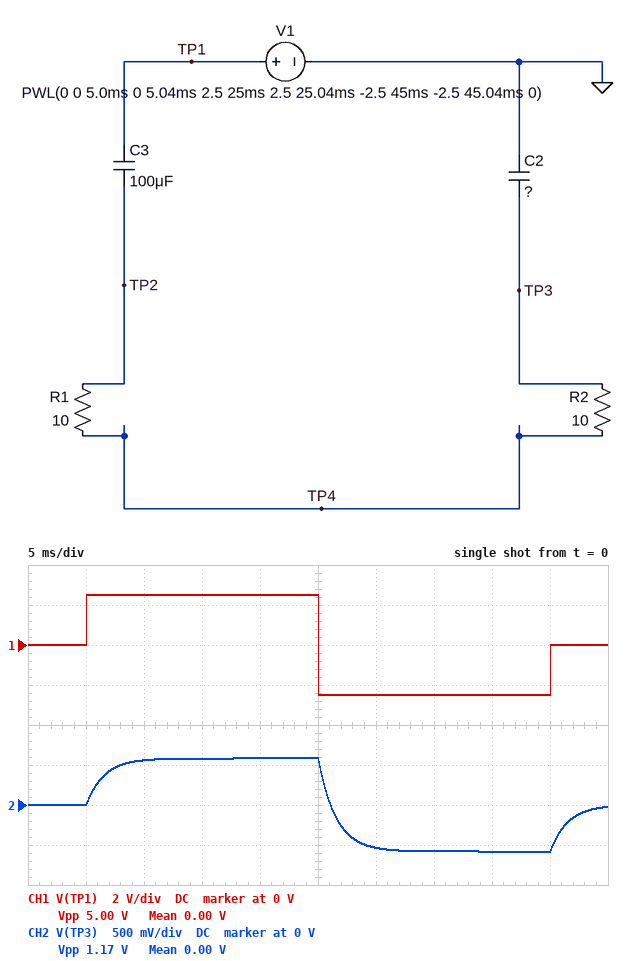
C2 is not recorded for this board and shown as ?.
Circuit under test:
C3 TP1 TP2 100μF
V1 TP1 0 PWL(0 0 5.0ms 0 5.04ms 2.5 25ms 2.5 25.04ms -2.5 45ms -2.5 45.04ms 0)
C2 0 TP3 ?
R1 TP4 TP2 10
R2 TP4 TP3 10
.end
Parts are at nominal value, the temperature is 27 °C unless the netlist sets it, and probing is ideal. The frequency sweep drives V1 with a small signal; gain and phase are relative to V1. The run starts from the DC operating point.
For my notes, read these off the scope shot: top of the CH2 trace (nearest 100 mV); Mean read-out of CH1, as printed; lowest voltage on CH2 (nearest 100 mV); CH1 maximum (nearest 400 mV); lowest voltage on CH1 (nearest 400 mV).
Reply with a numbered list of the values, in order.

1. 600 mV
2. 0.00 V
3. -600 mV
4. 2.4 V
5. -2.4 V
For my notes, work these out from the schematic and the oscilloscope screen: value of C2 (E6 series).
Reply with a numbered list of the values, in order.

1. 330 µF
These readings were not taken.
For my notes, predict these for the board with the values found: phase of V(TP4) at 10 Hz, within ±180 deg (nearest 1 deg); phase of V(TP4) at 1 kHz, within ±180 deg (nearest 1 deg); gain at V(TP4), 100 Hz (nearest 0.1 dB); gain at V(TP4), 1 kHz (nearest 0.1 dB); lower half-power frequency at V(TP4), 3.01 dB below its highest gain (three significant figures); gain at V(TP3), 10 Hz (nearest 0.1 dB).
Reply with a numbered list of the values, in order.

1. 6 deg
2. 3 deg
3. -8.3 dB
4. -6.1 dB
5. 78.1 Hz
6. -12.7 dB
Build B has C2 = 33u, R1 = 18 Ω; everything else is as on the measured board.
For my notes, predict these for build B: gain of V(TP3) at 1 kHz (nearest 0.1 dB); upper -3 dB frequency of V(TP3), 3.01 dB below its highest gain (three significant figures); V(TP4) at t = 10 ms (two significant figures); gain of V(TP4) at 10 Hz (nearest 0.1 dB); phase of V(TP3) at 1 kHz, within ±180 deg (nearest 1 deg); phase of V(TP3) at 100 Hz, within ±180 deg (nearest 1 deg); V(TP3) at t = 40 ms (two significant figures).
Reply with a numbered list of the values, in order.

1. -15.5 dB
2. 229 Hz
3. 1.9 V
4. -2.5 dB
5. -77 deg
6. -24 deg
7. -1.9 V
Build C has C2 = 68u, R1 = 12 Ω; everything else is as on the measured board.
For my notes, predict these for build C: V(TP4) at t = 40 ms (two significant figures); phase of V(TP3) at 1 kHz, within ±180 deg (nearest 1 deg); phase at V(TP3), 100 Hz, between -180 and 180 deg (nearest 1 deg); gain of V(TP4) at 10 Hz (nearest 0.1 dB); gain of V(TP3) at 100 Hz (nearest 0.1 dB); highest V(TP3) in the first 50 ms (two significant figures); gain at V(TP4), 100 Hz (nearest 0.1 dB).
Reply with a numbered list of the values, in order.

1. -1.5 V
2. -80 deg
3. -29 deg
4. -4.5 dB
5. -5.7 dB
6. 1.5 V
7. -5.0 dB
